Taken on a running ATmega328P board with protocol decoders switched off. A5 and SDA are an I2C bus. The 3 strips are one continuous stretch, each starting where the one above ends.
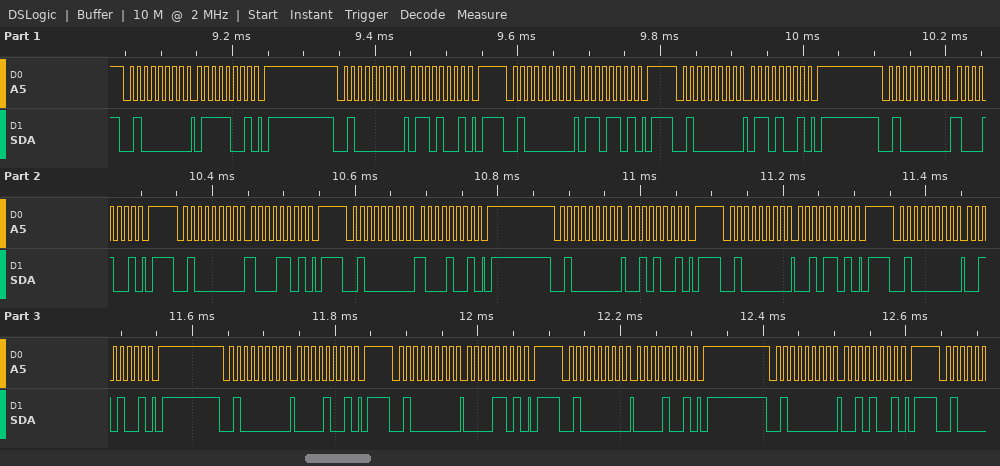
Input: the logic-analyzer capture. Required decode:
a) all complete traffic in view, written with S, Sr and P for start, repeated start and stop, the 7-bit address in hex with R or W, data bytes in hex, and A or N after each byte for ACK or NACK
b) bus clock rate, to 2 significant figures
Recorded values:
S 20W A 79 A P S 20W A 69 A P S 20W A 6D A P S 20W A 69 A P S 20W A 89 A P S 20W A 8D A P S 20W A 89 A P S 20W A 29 A P S 20W A 2D A P S 20W A 29 A P S 20W A 09 A P S 20W A 0D A P S 20W A 09 A P S 20W A 29 A P
100 kHz
